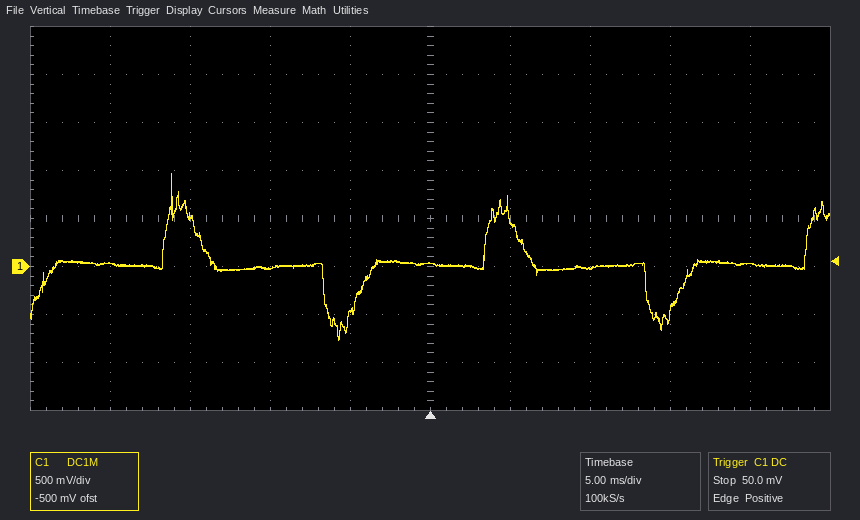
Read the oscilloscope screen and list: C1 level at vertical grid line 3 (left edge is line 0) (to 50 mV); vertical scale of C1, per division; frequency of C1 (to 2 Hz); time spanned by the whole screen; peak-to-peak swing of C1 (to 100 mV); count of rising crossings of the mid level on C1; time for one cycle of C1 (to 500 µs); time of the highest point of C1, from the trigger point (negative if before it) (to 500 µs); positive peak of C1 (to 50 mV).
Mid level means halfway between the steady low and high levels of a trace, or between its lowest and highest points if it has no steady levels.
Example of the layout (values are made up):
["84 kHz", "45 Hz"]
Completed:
["0 mV", "500 mV", "50 Hz", "50 ms", "1.70 V", "3", "20.0 ms", "-16.0 ms", "950 mV"]
